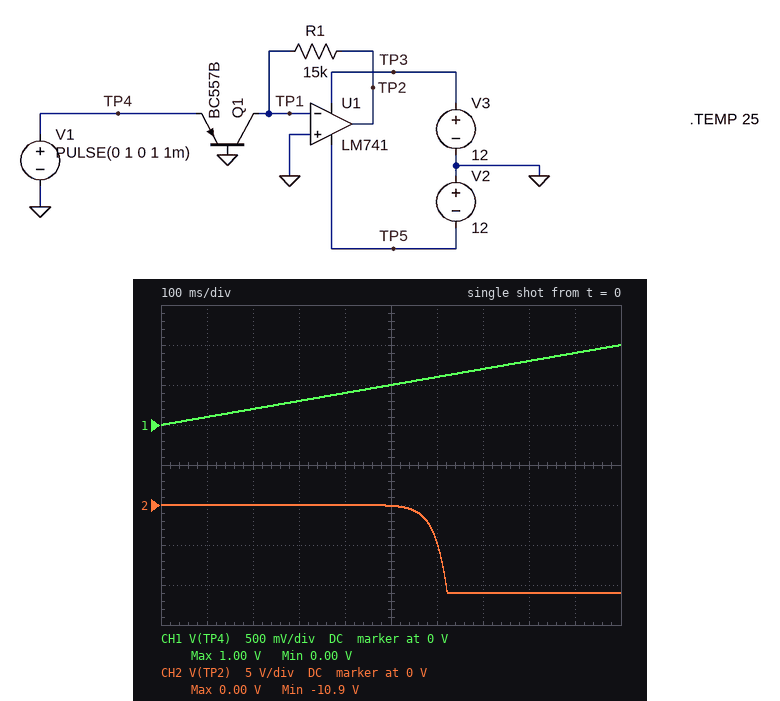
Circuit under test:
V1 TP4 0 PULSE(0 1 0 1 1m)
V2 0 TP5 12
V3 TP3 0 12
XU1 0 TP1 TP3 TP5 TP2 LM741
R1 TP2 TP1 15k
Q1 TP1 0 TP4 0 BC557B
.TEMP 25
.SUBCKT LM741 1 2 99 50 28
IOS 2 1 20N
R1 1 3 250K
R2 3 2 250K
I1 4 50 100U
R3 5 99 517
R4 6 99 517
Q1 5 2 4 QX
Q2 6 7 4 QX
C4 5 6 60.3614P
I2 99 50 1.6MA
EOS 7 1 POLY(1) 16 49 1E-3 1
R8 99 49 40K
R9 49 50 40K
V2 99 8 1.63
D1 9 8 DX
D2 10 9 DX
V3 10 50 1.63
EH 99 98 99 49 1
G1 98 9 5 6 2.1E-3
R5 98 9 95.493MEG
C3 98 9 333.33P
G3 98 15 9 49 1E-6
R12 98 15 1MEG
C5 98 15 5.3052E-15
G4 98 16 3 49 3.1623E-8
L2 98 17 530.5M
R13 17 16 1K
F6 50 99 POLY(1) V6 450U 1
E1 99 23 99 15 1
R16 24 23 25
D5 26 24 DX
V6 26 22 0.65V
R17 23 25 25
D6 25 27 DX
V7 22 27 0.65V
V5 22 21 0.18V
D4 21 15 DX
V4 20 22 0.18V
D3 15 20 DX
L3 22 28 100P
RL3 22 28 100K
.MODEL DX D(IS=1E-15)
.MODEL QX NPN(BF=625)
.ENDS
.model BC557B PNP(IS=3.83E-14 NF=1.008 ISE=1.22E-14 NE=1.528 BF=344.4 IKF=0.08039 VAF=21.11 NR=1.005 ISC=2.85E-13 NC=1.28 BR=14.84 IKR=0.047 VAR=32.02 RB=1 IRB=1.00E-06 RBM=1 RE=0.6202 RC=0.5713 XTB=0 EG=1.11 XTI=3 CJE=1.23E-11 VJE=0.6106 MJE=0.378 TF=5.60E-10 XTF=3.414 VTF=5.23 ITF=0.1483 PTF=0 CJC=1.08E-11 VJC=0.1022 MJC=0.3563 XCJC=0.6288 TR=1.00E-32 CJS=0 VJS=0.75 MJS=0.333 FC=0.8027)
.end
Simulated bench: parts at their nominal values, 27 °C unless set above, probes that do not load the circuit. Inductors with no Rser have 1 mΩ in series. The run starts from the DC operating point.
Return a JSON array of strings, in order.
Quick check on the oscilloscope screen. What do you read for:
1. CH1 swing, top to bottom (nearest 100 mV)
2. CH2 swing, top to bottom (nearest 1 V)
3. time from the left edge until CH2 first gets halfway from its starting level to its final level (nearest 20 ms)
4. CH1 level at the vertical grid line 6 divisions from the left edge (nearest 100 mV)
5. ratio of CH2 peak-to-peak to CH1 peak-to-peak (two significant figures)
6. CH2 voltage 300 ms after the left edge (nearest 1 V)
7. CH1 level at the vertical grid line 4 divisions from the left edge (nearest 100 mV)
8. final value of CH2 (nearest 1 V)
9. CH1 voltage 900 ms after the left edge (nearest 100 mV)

["1.0 V", "11 V", "600 ms", "600 mV", "11", "0 V", "400 mV", "-11 V", "900 mV"]
